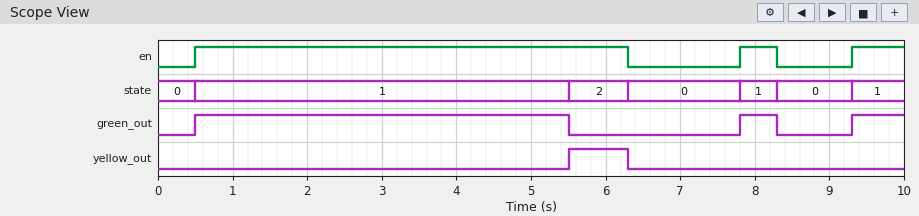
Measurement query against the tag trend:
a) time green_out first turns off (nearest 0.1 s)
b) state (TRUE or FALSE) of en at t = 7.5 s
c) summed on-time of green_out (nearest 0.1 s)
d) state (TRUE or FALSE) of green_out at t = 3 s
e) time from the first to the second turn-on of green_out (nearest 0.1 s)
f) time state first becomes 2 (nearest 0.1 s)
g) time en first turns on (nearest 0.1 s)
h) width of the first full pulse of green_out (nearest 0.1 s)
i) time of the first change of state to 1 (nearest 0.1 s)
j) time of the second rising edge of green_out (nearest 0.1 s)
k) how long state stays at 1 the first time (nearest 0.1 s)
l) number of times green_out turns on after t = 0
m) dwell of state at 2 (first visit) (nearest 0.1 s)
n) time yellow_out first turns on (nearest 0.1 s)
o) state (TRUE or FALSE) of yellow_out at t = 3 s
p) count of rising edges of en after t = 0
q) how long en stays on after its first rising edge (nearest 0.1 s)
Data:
5.5 s
FALSE
6.2 s
TRUE
7.3 s
5.5 s
0.5 s
5.0 s
0.5 s
7.8 s
5.0 s
3
0.8 s
5.5 s
FALSE
3
5.8 s
